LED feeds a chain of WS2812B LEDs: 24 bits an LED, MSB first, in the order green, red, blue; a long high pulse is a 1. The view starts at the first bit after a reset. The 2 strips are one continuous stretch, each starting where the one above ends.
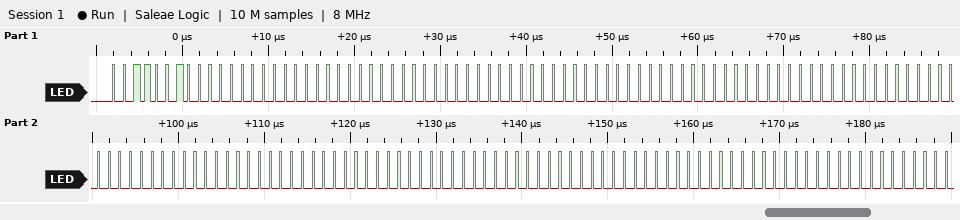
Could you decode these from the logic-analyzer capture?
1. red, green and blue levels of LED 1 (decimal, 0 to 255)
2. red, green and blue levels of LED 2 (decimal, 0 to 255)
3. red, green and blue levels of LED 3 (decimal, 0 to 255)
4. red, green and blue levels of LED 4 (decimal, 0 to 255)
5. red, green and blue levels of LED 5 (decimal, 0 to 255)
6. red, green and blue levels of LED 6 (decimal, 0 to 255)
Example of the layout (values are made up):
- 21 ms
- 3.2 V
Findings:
- 0, 50, 0
- 0, 0, 0
- 0, 0, 0
- 0, 0, 0
- 0, 0, 0
- 0, 0, 0
